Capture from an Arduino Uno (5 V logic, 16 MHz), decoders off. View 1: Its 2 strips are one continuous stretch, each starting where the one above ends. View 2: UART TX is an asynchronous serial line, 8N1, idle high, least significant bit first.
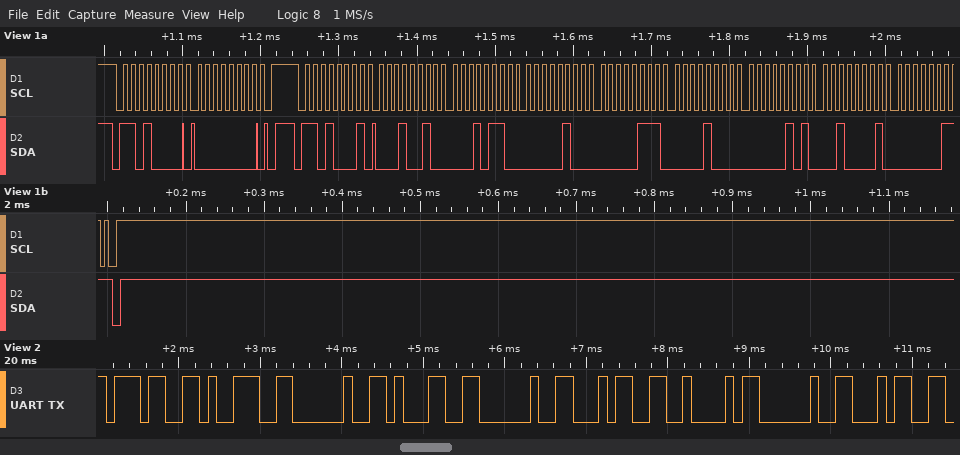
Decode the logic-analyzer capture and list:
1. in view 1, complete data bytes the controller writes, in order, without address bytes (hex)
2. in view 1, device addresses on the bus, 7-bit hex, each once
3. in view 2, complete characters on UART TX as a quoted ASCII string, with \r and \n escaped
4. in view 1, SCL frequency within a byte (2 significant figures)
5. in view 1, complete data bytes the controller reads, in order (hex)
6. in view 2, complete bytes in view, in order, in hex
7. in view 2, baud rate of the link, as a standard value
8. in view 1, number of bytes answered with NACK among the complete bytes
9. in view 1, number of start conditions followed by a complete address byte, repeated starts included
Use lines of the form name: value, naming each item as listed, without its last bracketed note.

in view 1, complete data bytes the controller writes, in order, without address bytes: 00
in view 1, device addresses on the bus, 7-bit hex, each once: 0x68
in view 2, complete characters on UART TX as a quoted ASCII string, with \r and \n escaped: "79 1 4B 4"
in view 1, SCL frequency within a byte: 100 kHz
in view 1, complete data bytes the controller reads, in order: 12 16 04 07 08 05 21 03
in view 2, complete bytes in view, in order, in hex: 37 39 20 31 20 34 42 20 34
in view 2, baud rate of the link, as a standard value: 9600 baud
in view 1, number of bytes answered with NACK among the complete bytes: 1
in view 1, number of start conditions followed by a complete address byte, repeated starts included: 2
